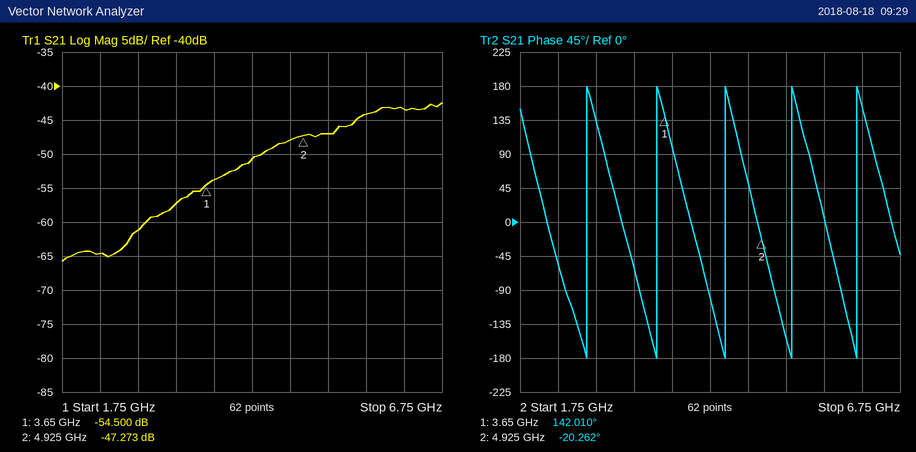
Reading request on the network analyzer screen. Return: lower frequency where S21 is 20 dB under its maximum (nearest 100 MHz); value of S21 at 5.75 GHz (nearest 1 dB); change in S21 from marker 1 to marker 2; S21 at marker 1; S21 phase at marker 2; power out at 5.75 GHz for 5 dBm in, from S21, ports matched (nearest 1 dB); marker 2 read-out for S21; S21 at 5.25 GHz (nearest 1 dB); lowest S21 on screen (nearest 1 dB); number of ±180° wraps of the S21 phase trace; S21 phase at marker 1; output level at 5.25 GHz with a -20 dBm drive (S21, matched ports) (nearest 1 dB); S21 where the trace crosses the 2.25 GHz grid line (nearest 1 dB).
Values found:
2.6 GHz
-44 dB
7.227 dB
-54.500 dB
-20.262°
-39 dBm
-47.273 dB
-47 dB
-66 dB
5
142.010°
-67 dBm
-65 dB
